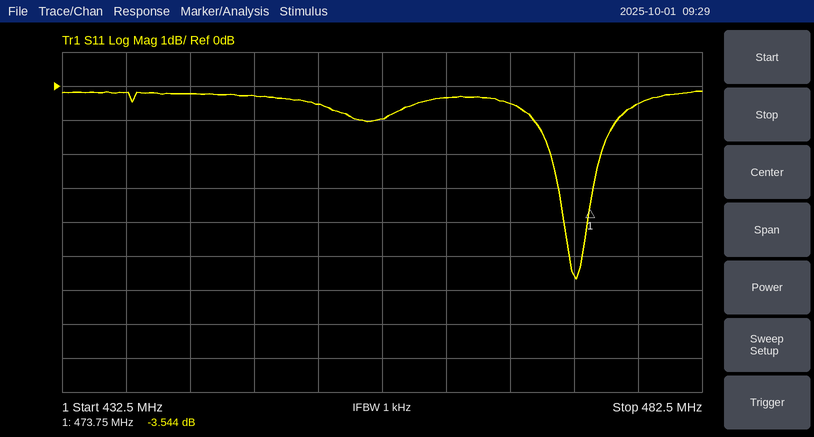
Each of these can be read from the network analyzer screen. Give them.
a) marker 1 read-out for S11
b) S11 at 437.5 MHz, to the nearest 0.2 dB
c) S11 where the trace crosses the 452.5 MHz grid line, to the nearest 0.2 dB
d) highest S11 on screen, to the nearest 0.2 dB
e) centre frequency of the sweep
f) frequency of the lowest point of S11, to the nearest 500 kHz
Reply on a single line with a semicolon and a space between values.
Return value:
-3.544 dB; -0.2 dB; -0.6 dB; -0.2 dB; 457.5 MHz; 472.5 MHz
